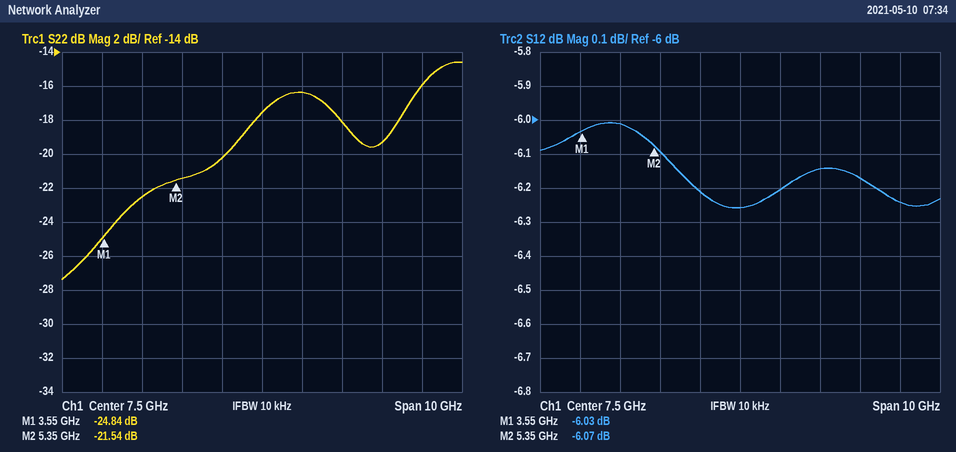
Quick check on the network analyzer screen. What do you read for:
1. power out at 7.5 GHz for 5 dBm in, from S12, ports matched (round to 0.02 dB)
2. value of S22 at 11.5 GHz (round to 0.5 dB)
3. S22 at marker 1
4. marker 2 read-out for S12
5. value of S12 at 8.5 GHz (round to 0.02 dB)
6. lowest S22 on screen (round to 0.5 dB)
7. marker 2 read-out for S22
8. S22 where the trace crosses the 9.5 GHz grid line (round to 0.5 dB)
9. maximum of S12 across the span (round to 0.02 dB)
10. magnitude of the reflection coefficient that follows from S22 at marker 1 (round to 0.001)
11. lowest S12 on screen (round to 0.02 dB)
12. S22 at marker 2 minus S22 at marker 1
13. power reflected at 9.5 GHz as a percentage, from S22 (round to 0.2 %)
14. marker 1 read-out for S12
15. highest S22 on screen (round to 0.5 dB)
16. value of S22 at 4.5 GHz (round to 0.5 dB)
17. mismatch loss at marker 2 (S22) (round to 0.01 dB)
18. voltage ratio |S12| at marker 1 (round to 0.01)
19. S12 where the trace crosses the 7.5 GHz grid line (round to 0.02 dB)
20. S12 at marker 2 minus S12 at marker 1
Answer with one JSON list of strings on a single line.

["-1.26 dBm", "-16.0 dB", "-24.84 dB", "-6.07 dB", "-6.20 dB", "-27.5 dB", "-21.54 dB", "-18.0 dB", "-6.00 dB", "0.057", "-6.26 dB", "3.30 dB", "1.6 %", "-6.03 dB", "-14.5 dB", "-22.5 dB", "0.03 dB", "0.50", "-6.26 dB", "-0.04 dB"]
